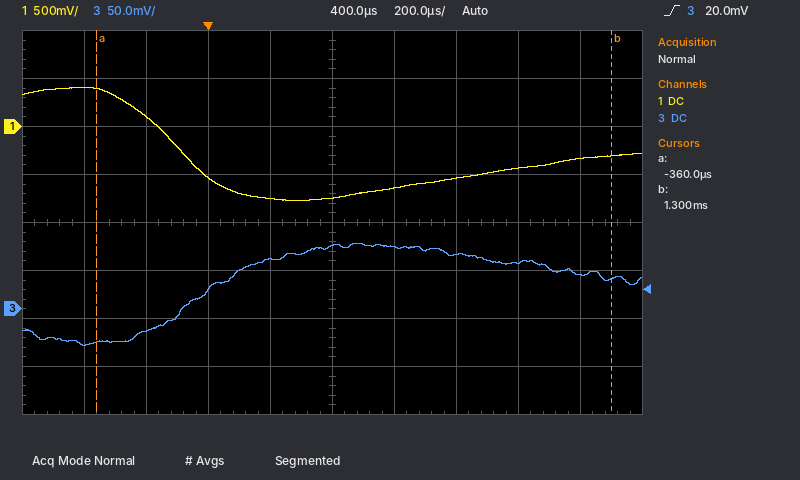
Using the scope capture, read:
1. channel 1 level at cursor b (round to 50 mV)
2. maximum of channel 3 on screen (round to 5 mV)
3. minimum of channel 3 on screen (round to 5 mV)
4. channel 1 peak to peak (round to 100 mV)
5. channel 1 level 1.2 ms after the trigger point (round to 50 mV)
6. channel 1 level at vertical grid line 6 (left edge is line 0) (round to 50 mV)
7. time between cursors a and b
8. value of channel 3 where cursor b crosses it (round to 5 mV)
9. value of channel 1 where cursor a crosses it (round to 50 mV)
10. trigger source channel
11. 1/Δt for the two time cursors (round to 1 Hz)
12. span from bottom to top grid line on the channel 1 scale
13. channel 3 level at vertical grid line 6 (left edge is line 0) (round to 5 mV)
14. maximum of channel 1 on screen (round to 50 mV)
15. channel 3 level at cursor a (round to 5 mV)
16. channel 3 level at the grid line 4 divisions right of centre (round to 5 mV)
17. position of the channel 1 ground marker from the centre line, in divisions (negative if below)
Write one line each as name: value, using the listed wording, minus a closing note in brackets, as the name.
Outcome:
channel 1 level at cursor b: -300 mV
maximum of channel 3 on screen: 70 mV
minimum of channel 3 on screen: -40 mV
channel 1 peak to peak: 1.20 V
channel 1 level 1.2 ms after the trigger point: -350 mV
channel 1 level at vertical grid line 6 (left edge is line 0): -650 mV
time between cursors a and b: 1.66 ms
value of channel 3 where cursor b crosses it: 30 mV
value of channel 1 where cursor a crosses it: 400 mV
trigger source channel: channel 3
1/Δt for the two time cursors: 602 Hz
span from bottom to top grid line on the channel 1 scale: 4 V
channel 3 level at vertical grid line 6 (left edge is line 0): 65 mV
maximum of channel 1 on screen: 400 mV
channel 3 level at cursor a: -35 mV
channel 3 level at the grid line 4 divisions right of centre: 35 mV
position of the channel 1 ground marker from the centre line, in divisions: +2.0 div
